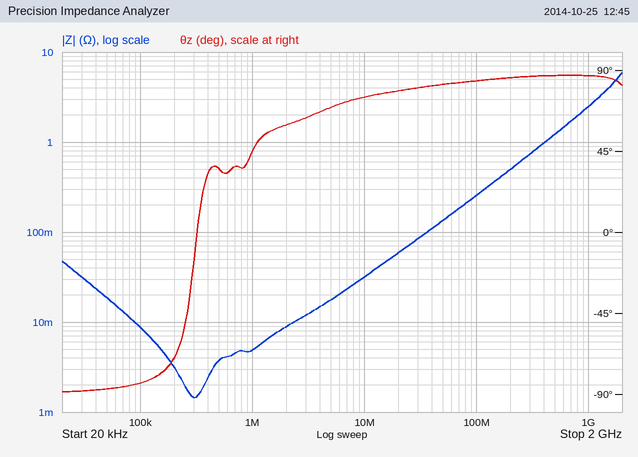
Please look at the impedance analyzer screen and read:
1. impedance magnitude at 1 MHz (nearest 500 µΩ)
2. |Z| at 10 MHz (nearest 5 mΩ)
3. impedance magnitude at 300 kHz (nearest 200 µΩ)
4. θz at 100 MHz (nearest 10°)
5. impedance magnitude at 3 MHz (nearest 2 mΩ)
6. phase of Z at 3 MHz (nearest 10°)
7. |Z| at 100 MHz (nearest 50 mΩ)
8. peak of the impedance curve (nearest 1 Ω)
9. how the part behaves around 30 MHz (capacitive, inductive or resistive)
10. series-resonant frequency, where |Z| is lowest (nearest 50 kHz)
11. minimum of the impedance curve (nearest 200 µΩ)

5.0 mΩ
30 mΩ
1.4 mΩ
80°
12 mΩ
60°
250 mΩ
6 Ω
inductive
300 kHz
1.4 mΩ
